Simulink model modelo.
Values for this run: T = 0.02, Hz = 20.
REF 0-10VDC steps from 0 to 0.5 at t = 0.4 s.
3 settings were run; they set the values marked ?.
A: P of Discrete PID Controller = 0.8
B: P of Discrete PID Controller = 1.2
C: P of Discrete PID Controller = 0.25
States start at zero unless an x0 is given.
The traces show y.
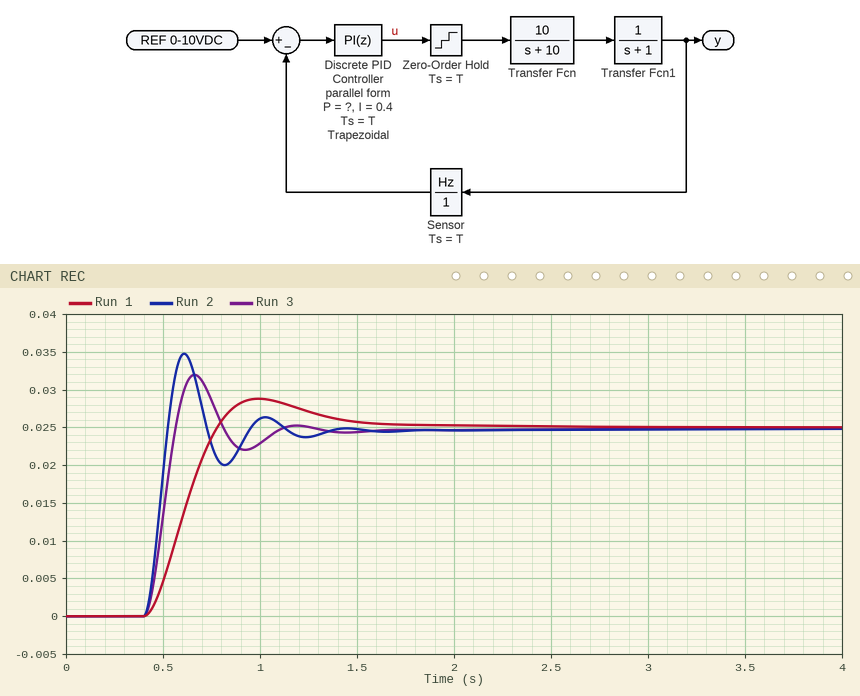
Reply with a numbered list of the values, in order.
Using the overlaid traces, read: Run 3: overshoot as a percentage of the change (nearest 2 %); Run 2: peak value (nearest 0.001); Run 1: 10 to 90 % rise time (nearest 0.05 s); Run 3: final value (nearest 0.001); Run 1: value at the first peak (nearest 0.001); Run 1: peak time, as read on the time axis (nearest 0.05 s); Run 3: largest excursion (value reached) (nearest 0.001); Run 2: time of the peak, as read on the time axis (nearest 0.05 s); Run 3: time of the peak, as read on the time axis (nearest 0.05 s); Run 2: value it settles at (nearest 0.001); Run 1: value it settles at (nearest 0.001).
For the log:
1. 28 %
2. 0.035
3. 0.25 s
4. 0.025
5. 0.029
6. 1.00 s
7. 0.032
8. 0.60 s
9. 0.65 s
10. 0.025
11. 0.025
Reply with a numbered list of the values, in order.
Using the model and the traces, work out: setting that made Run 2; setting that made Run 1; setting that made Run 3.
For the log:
1. B
2. C
3. A
